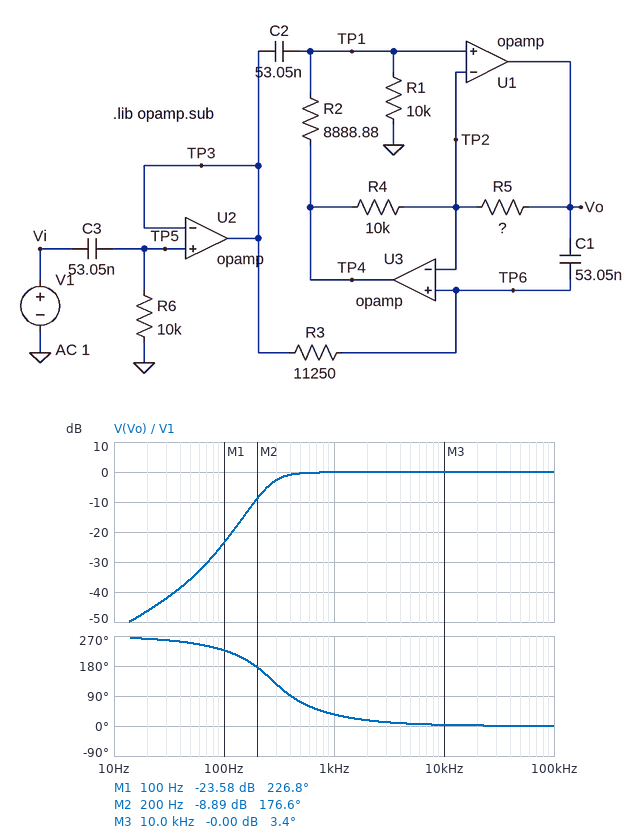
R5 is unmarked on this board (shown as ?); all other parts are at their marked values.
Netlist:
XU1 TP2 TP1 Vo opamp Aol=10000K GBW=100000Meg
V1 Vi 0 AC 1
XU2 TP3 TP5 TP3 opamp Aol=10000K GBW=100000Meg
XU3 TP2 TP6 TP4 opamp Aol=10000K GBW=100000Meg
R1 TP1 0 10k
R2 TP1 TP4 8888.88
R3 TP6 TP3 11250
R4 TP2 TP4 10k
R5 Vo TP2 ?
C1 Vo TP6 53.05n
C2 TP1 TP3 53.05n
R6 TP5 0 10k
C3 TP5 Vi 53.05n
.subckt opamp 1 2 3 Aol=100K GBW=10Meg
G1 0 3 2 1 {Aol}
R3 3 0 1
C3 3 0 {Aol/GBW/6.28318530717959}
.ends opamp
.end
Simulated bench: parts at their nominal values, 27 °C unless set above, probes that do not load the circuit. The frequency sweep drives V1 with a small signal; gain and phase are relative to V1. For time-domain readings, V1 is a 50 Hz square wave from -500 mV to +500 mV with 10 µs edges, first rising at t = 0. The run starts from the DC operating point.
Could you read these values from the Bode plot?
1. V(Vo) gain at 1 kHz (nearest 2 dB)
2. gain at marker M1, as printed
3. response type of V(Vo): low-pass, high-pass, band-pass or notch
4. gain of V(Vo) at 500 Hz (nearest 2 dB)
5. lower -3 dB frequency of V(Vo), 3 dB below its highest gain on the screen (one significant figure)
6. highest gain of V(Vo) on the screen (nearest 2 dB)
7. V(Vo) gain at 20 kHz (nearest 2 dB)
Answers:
0 dB
-23.58 dB
high-pass
0 dB
300 Hz
0 dB
0 dB
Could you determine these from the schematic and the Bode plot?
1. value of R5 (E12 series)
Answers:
12 kΩ
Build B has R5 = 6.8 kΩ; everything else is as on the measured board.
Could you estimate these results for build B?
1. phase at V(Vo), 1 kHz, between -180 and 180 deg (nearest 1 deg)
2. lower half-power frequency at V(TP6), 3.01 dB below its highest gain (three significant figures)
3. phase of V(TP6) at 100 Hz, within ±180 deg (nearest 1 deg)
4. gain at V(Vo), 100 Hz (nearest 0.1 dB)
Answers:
36 deg
605 Hz
58 deg
-19.5 dB
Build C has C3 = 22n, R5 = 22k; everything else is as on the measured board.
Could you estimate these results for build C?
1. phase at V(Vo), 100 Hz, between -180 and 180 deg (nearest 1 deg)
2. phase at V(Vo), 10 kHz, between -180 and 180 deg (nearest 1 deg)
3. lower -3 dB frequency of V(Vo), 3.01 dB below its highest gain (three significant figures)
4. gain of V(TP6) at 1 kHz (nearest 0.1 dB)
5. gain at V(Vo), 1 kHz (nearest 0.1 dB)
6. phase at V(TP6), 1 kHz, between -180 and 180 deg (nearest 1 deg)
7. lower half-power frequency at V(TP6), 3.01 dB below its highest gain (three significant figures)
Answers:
-142 deg
6 deg
623 Hz
-2.2 dB
-1.5 dB
53 deg
837 Hz
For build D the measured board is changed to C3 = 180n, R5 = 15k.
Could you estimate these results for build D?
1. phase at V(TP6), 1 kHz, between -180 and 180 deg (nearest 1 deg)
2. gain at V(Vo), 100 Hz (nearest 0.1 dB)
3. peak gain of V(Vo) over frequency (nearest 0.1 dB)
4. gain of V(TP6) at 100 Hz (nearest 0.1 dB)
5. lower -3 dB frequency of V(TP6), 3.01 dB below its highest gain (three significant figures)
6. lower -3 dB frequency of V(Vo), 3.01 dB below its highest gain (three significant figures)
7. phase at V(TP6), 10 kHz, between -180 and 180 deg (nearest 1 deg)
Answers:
23 deg
-8.3 dB
1.1 dB
-3.8 dB
446 Hz
185 Hz
2 deg
